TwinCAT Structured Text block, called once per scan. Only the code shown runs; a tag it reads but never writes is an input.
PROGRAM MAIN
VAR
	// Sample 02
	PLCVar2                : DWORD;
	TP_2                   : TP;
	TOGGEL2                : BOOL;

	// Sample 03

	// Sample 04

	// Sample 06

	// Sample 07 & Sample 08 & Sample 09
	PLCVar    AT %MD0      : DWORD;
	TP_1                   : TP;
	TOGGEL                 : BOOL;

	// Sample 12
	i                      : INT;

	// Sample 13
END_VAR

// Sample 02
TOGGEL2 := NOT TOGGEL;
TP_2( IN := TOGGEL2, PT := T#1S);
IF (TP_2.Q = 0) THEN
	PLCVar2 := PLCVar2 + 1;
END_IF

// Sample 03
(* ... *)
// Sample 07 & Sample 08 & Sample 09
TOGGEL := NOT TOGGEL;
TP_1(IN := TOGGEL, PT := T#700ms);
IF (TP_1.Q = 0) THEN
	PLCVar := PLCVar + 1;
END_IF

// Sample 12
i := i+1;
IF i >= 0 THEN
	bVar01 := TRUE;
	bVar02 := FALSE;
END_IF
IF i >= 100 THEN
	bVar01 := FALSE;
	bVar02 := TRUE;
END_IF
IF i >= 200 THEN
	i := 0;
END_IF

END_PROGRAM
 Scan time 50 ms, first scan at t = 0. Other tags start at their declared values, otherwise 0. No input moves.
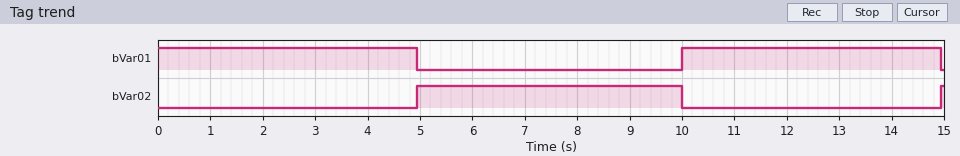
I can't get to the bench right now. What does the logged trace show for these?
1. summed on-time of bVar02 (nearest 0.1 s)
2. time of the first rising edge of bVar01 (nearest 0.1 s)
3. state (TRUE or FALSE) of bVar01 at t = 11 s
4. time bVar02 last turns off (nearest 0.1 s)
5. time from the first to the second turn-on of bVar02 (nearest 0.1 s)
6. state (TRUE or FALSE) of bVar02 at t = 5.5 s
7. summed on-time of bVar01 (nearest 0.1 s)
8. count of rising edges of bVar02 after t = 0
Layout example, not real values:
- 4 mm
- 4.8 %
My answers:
- 5.1 s
- 10.0 s
- TRUE
- 10.0 s
- 10.0 s
- TRUE
- 9.9 s
- 2
